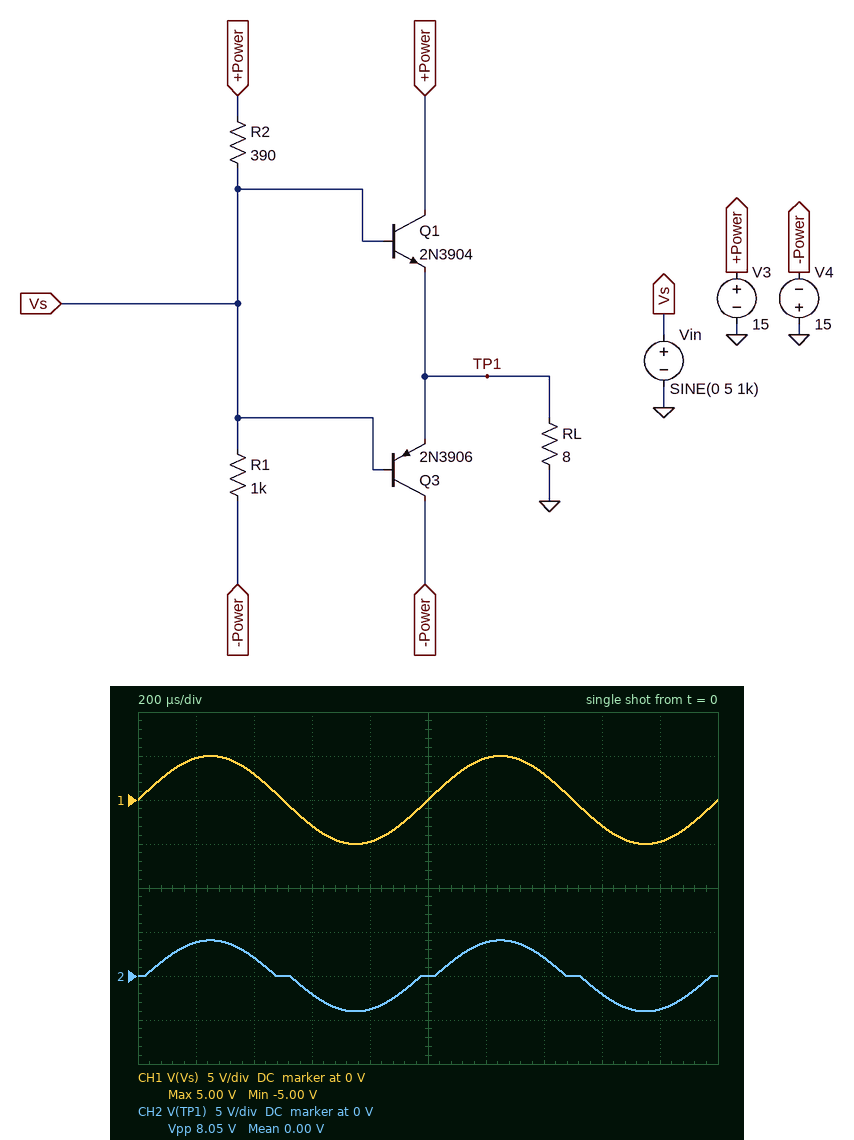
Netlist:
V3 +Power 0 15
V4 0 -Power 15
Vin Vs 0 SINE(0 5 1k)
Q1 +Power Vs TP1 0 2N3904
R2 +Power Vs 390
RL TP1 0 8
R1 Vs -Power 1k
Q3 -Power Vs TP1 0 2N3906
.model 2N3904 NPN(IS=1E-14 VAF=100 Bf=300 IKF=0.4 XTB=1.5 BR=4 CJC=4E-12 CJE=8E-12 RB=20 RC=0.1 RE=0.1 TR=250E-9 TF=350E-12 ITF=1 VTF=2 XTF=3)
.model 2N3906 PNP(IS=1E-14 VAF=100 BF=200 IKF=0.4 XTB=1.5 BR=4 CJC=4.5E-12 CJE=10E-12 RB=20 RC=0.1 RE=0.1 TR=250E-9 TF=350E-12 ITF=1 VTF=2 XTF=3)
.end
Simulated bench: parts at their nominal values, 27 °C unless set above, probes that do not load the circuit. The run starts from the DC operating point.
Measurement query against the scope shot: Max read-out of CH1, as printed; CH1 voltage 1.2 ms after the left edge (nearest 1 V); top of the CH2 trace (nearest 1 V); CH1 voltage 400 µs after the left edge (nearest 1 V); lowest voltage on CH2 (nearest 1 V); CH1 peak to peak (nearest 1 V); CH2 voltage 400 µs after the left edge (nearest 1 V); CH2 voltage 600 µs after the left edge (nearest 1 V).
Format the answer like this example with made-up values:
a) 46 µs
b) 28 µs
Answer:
a) 5.00 V
b) 5 V
c) 4 V
d) 3 V
e) -4 V
f) 10 V
g) 2 V
h) -2 V
